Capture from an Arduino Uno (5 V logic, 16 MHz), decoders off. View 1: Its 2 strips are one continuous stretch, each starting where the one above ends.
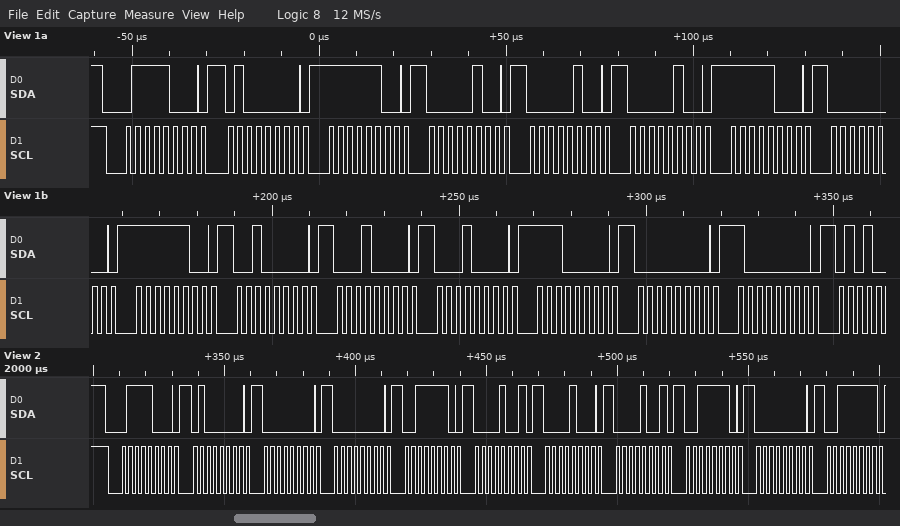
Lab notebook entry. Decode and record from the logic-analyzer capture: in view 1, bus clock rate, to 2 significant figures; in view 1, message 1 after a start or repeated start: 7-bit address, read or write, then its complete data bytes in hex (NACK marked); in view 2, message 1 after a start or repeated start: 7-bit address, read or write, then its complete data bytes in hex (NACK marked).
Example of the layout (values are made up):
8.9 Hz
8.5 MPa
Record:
400 kHz
0x3C write: 40 FC 04 04 04 F8 00 FC 20 10 10 E0 00 80
0x3C write: 40 00 00 3E 09 08 09 3E 00 3F
